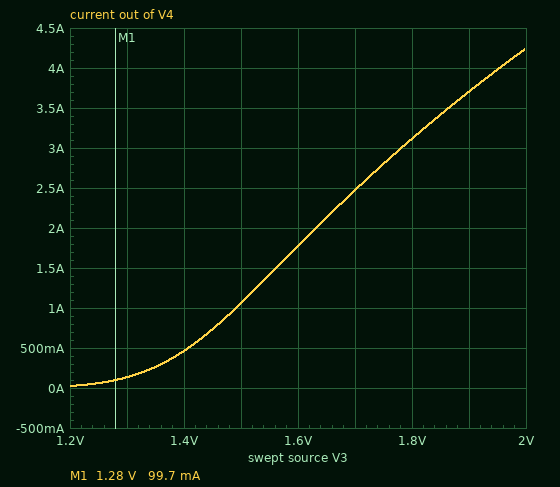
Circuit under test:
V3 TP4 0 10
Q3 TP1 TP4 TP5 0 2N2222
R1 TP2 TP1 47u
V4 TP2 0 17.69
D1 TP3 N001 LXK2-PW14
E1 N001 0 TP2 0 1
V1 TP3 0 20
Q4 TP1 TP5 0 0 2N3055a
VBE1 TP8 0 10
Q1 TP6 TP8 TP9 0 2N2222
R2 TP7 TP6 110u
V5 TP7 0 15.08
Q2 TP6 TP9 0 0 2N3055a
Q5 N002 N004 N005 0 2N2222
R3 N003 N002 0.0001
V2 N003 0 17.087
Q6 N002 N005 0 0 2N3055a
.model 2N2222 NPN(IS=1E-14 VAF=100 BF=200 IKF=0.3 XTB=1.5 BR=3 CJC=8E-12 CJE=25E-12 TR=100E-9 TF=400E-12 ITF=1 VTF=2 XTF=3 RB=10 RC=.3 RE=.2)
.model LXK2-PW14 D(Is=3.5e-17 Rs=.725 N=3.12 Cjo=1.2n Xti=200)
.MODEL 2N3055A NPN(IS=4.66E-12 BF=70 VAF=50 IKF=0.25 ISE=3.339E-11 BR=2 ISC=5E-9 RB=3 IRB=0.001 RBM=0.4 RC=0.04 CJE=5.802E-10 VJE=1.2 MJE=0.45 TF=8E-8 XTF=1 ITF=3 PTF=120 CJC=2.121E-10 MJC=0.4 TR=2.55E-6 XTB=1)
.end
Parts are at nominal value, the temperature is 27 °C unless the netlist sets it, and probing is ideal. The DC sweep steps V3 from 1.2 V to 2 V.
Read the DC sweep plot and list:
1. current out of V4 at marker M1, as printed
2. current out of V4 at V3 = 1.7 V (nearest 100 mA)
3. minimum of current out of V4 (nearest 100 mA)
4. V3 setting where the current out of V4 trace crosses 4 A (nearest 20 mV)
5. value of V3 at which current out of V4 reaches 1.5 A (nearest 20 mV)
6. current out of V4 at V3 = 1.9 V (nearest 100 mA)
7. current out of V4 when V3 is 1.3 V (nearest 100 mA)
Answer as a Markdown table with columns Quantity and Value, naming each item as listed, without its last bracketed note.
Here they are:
| Quantity | Value |
|---|---|
| current out of V4 at marker M1, as printed | 99.7 mA |
| current out of V4 at V3 = 1.7 V | 2.5 A |
| minimum of current out of V4 | 0 A |
| V3 setting where the current out of V4 trace crosses 4 A | 1.96 V |
| value of V3 at which current out of V4 reaches 1.5 A | 1.56 V |
| current out of V4 at V3 = 1.9 V | 3.7 A |
| current out of V4 when V3 is 1.3 V | 100 mA |
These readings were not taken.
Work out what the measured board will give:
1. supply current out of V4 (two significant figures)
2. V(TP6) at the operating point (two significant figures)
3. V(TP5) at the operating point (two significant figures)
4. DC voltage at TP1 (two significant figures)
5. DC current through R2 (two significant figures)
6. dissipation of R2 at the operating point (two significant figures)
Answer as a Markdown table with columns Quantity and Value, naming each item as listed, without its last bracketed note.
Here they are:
| Quantity | Value |
|---|---|
| supply current out of V4 | 19 A |
| V(TP6) at the operating point | 15 V |
| V(TP5) at the operating point | 3.4 V |
| DC voltage at TP1 | 18 V |
| DC current through R2 | 18 A |
| dissipation of R2 at the operating point | 36 mW |
